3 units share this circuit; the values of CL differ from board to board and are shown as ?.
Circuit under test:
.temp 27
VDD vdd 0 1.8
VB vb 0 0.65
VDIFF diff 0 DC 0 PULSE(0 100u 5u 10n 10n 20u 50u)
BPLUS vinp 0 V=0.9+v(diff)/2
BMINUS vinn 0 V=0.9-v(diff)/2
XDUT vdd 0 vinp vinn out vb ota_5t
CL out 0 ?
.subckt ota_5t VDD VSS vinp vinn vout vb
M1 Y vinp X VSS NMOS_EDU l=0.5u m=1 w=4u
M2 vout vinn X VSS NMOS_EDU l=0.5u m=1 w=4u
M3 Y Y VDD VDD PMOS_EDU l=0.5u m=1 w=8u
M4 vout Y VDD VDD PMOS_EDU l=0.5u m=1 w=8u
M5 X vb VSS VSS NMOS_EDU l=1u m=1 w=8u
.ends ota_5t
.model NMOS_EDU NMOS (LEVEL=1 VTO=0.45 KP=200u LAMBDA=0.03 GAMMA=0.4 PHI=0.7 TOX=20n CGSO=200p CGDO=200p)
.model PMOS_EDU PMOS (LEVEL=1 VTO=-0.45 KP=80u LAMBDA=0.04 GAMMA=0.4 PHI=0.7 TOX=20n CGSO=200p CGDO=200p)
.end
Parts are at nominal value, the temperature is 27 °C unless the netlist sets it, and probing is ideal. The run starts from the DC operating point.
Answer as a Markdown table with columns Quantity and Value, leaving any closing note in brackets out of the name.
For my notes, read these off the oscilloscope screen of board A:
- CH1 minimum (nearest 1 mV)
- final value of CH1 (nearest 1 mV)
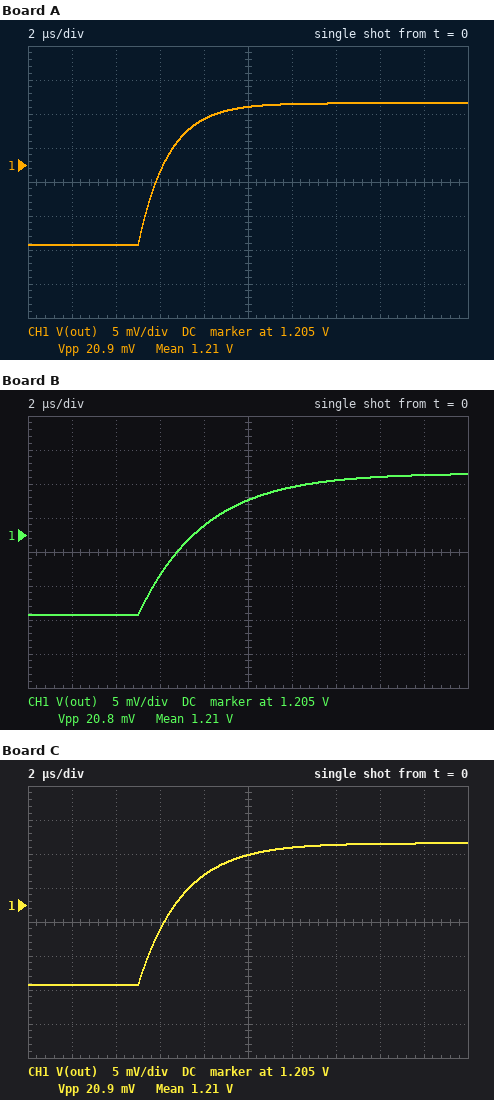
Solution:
| Quantity | Value |
|---|---|
| CH1 minimum | 1.193 V |
| final value of CH1 | 1.214 V |
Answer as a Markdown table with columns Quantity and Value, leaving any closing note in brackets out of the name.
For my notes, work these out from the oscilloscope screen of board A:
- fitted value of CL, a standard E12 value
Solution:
| Quantity | Value |
|---|---|
| fitted value of CL, a standard E12 value | 1.5 pF |
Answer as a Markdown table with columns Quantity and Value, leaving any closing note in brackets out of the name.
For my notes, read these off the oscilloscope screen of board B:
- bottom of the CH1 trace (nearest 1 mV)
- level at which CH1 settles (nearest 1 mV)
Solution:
| Quantity | Value |
|---|---|
| bottom of the CH1 trace | 1.193 V |
| level at which CH1 settles | 1.214 V |
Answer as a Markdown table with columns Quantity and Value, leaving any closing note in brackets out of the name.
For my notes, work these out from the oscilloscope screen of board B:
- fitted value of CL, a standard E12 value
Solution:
| Quantity | Value |
|---|---|
| fitted value of CL, a standard E12 value | 3.3 pF |
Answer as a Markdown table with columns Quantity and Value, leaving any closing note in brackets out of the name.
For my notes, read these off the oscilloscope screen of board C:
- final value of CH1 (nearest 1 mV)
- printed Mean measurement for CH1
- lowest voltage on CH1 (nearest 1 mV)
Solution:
| Quantity | Value |
|---|---|
| final value of CH1 | 1.214 V |
| printed Mean measurement for CH1 | 1.21 V |
| lowest voltage on CH1 | 1.193 V |
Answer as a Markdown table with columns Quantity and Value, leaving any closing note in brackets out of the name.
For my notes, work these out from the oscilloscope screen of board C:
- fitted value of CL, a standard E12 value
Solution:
| Quantity | Value |
|---|---|
| fitted value of CL, a standard E12 value | 2.2 pF |
